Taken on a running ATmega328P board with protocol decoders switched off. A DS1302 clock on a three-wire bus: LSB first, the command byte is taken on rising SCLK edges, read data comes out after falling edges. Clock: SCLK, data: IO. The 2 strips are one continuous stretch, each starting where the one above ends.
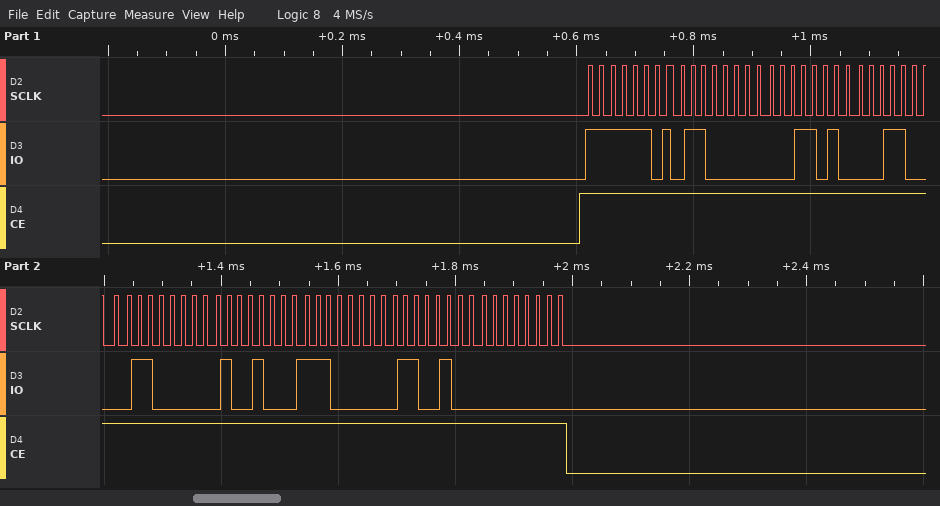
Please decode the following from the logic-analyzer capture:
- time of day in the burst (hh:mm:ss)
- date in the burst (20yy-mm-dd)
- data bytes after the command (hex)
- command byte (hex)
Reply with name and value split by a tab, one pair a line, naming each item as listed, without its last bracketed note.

time of day in the burst	18:58:06
date in the burst	2026-12-06
data bytes after the command	06 58 18 06 12 07 26 00
command byte	0xBF
